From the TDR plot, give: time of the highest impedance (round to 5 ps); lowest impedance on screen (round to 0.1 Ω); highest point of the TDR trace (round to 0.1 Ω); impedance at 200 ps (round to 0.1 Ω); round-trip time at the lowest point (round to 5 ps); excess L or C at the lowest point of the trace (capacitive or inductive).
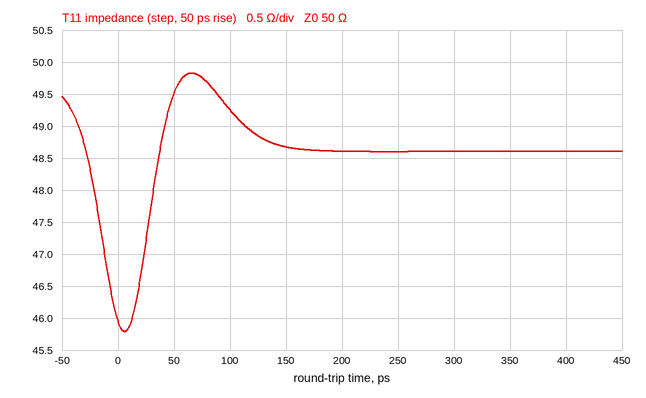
65 ps
45.8 Ω
49.8 Ω
48.6 Ω
5 ps
capacitive
